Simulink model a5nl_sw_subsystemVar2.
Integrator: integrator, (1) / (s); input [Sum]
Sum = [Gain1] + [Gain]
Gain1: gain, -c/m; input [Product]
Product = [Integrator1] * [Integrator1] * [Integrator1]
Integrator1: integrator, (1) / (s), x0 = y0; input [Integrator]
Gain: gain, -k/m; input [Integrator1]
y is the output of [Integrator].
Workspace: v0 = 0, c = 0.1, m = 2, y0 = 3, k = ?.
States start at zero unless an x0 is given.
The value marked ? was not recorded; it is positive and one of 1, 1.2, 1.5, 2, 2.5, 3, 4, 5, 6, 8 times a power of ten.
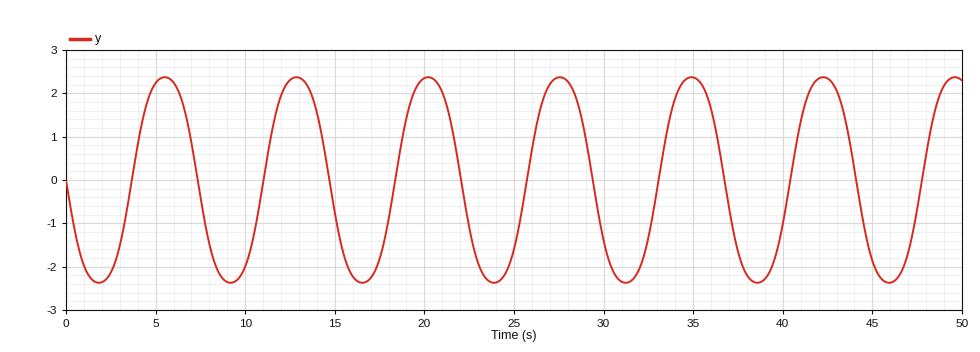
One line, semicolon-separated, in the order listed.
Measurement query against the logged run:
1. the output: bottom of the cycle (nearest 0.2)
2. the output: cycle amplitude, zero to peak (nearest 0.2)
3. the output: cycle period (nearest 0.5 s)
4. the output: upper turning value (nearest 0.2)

-2.4; 2.4; 7.5 s; 2.4
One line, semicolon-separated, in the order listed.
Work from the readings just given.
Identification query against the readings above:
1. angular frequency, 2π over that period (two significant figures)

0.84 rad/s
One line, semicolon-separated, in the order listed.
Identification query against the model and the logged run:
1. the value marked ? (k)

0.8
